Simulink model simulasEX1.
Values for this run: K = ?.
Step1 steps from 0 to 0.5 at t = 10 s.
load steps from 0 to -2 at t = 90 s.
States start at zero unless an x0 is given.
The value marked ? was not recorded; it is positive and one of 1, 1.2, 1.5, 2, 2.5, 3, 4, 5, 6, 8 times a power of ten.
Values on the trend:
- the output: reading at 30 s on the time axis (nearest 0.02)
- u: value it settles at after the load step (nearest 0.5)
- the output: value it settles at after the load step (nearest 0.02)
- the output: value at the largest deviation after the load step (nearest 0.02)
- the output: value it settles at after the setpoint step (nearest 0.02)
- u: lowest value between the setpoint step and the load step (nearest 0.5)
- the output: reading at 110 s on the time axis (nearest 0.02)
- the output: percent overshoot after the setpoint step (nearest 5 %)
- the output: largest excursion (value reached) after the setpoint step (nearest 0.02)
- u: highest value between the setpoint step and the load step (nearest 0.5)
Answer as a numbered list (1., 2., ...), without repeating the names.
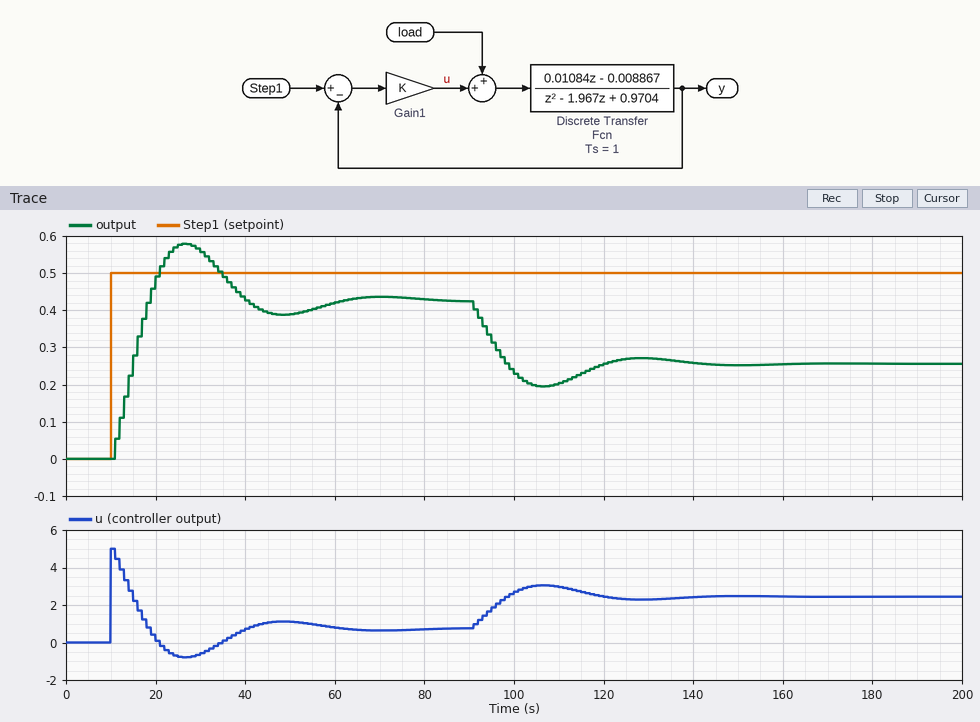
1. 0.56
2. 2.5
3. 0.26
4. 0.20
5. 0.42
6. -1.0
7. 0.20
8. 35 %
9. 0.58
10. 5.0
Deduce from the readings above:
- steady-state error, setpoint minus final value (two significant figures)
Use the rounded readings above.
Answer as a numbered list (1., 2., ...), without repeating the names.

1. 0.080
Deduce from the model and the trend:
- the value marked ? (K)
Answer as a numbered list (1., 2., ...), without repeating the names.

1. 10
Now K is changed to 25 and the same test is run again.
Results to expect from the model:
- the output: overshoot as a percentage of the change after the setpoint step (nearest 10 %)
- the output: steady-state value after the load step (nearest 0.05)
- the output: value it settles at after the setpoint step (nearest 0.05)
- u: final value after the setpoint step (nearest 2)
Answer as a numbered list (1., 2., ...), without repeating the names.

1. 30 %
2. 0.40
3. 0.45
4. 0
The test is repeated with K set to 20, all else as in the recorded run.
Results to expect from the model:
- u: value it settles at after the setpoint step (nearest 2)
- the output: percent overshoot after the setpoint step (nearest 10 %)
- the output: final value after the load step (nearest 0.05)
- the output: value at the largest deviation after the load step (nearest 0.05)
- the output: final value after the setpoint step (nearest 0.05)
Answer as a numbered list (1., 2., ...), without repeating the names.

1. 0
2. 30 %
3. 0.35
4. 0.35
5. 0.45
